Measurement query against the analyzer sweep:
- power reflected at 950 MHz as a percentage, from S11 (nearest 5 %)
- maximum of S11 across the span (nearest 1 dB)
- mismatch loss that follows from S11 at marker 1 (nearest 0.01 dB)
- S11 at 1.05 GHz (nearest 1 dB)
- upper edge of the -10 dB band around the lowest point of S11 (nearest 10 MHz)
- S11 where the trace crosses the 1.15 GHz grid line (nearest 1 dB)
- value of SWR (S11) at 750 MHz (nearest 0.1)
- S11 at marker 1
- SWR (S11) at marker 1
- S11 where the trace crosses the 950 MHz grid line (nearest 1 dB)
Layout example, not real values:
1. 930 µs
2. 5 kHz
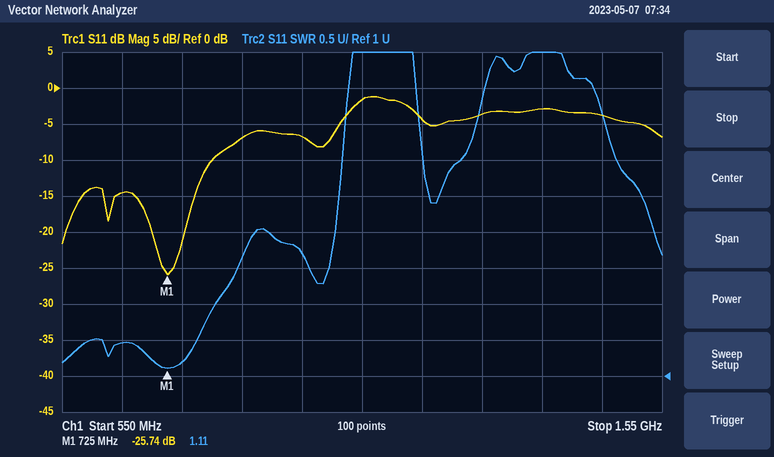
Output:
1. 20 %
2. -1 dB
3. 0.01 dB
4. -2 dB
5. 800 MHz
6. -4 dB
7. 1.2
8. -25.74 dB
9. 1.11
10. -7 dB
